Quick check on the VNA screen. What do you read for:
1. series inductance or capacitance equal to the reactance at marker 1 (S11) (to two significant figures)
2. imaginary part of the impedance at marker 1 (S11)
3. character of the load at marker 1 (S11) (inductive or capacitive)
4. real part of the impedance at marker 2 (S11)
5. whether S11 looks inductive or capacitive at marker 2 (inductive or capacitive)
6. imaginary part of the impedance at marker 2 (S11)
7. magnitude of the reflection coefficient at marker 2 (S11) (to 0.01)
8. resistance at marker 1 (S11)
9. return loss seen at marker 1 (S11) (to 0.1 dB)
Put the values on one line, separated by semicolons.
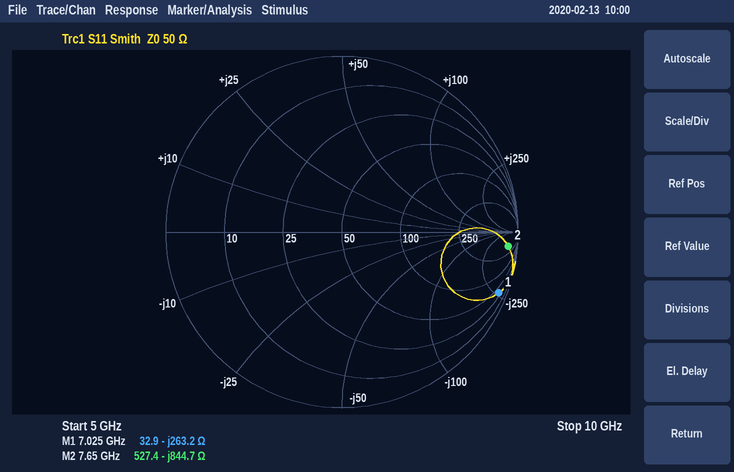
86 fF; -263.2 Ω; capacitive; 527.4 Ω; capacitive; -844.7 Ω; 0.95; 32.9 Ω; 0.4 dB
